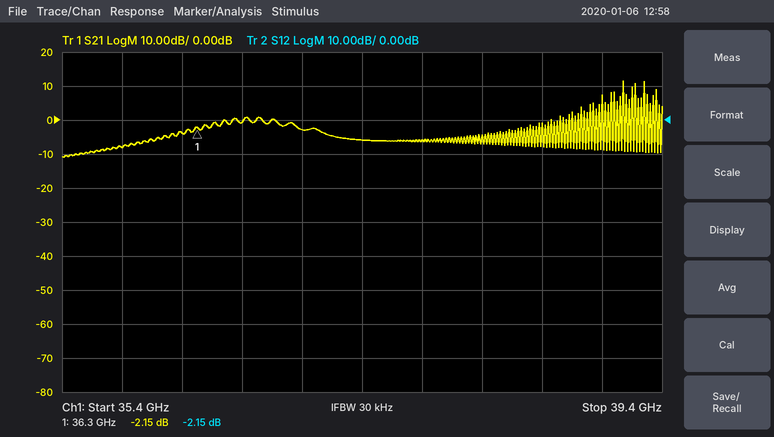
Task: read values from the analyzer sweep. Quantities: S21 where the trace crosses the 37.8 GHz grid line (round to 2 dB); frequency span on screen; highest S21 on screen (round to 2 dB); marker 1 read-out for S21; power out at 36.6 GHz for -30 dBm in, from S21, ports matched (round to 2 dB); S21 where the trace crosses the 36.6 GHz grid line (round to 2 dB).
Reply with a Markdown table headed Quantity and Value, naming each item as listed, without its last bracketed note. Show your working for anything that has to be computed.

| Quantity | Value |
|---|---|
| S21 where the trace crosses the 37.8 GHz grid line | -6 dB |
| frequency span on screen | 4 GHz |
| highest S21 on screen | 12 dB |
| marker 1 read-out for S21 | -2.15 dB |
| power out at 36.6 GHz for -30 dBm in, from S21, ports matched | -30 dBm + (0 dB) = -30 dBm |
| S21 where the trace crosses the 36.6 GHz grid line | 0 dB |
